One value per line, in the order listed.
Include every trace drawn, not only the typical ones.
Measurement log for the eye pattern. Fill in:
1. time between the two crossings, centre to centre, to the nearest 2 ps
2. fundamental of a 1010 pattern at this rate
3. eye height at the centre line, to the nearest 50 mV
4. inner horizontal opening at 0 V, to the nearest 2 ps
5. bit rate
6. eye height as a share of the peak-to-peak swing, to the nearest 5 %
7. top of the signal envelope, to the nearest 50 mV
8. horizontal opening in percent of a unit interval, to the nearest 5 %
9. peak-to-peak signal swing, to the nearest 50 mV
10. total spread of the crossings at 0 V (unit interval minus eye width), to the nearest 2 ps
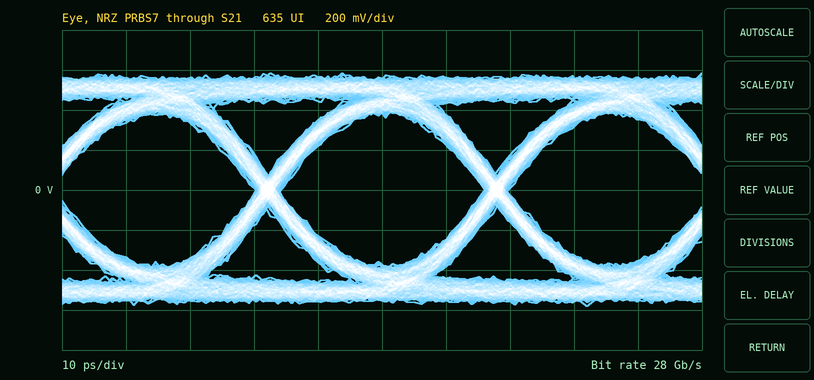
36 ps
14 GHz
750 mV
32 ps
28 Gb/s
65 %
600 mV
90 %
1.15 V
4 ps
